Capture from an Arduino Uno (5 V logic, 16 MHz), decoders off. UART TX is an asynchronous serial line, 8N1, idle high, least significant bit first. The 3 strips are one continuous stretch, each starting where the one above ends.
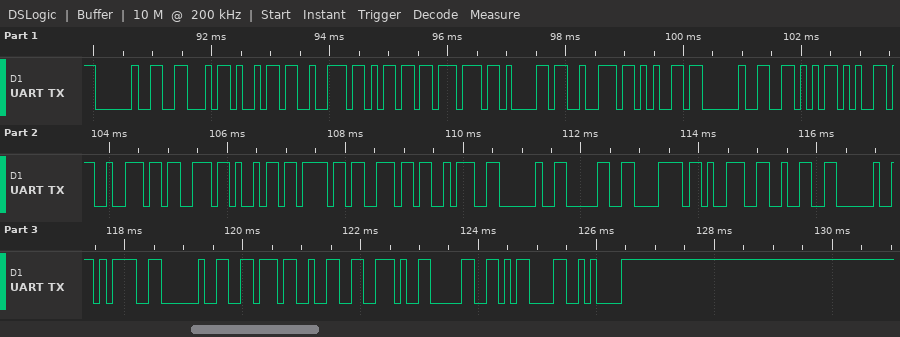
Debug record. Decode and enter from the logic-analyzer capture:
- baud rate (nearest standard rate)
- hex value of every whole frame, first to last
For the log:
9600 baud
20 46 69 72 6D 77 61 72 65 20 56 65 72 73 69 6F 6E 3A 20 30 78 39 32 20 3D 20 76 32 2E 30 0D 0A
